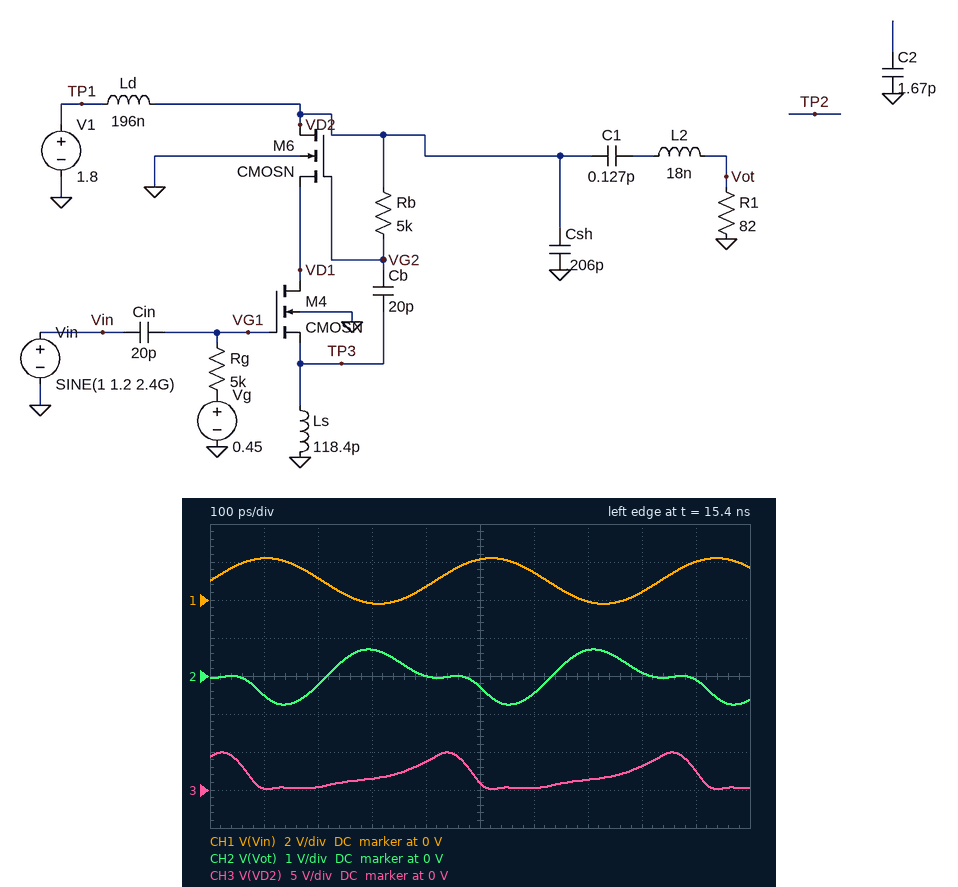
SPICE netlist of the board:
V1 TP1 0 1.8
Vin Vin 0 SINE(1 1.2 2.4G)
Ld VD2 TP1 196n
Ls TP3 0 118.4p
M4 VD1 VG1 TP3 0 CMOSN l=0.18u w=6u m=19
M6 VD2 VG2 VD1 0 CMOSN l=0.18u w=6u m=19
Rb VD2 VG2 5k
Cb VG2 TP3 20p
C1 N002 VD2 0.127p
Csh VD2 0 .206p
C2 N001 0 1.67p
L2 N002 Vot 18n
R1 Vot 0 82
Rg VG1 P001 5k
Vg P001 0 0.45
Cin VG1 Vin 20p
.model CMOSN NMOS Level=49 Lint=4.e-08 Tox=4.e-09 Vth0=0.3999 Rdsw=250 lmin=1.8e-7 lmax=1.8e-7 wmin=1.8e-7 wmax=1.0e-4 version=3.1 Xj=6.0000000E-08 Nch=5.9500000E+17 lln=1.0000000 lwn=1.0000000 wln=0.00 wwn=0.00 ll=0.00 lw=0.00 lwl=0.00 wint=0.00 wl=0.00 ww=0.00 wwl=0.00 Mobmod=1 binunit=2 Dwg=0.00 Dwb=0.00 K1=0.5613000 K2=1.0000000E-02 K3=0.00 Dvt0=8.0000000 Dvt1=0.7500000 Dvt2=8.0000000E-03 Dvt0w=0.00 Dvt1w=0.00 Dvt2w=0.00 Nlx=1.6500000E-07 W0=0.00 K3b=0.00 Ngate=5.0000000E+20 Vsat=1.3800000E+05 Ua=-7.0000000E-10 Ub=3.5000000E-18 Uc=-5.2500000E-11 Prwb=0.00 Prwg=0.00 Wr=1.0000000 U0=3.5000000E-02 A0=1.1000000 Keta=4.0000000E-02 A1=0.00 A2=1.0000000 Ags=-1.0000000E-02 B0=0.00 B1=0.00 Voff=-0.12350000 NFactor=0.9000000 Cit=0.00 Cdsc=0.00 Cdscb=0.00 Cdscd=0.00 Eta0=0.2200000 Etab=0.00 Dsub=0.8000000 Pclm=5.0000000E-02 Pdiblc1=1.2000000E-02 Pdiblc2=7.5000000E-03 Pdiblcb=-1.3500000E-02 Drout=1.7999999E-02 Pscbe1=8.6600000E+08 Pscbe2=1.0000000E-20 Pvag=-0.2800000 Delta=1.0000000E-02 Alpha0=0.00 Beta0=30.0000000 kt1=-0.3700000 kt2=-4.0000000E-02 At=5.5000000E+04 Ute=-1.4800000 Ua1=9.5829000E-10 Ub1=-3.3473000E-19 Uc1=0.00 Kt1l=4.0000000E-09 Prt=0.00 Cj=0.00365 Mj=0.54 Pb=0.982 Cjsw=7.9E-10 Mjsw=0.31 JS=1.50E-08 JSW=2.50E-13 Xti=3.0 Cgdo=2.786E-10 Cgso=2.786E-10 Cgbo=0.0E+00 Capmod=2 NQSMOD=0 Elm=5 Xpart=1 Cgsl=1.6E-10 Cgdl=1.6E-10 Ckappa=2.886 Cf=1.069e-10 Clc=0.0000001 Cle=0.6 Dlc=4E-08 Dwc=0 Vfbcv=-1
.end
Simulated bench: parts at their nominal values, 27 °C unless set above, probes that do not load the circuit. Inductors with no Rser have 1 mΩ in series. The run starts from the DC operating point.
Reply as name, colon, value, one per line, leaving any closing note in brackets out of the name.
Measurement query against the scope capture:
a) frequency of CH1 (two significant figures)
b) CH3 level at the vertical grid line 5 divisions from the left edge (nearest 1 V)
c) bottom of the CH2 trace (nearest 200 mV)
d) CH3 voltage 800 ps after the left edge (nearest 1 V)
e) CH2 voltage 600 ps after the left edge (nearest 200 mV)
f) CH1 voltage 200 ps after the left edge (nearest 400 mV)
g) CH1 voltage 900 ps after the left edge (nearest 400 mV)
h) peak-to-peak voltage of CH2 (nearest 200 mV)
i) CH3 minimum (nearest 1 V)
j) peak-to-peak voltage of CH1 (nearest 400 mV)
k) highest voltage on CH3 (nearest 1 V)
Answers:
frequency of CH1: 2.4 GHz
CH3 level at the vertical grid line 5 divisions from the left edge: 1 V
bottom of the CH2 trace: -800 mV
CH3 voltage 800 ps after the left edge: 3 V
CH2 voltage 600 ps after the left edge: -400 mV
CH1 voltage 200 ps after the left edge: 1.2 V
CH1 voltage 900 ps after the left edge: 2.0 V
peak-to-peak voltage of CH2: 1.4 V
CH3 minimum: 0 V
peak-to-peak voltage of CH1: 2.4 V
highest voltage on CH3: 5 V
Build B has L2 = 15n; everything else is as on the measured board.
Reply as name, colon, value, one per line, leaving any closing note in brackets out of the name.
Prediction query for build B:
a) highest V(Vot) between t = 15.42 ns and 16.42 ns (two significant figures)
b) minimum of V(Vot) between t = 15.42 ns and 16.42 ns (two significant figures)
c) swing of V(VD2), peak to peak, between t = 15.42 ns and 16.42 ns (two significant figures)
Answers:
highest V(Vot) between t = 15.42 ns and 16.42 ns: 720 mV
minimum of V(Vot) between t = 15.42 ns and 16.42 ns: -860 mV
swing of V(VD2), peak to peak, between t = 15.42 ns and 16.42 ns: 5.0 V
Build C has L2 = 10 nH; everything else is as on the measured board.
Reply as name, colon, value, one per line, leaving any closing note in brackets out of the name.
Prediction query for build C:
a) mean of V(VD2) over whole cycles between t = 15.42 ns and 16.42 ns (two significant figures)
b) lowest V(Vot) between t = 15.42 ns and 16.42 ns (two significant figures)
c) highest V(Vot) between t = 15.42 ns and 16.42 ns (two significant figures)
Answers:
mean of V(VD2) over whole cycles between t = 15.42 ns and 16.42 ns: 1.8 V
lowest V(Vot) between t = 15.42 ns and 16.42 ns: -1.3 V
highest V(Vot) between t = 15.42 ns and 16.42 ns: 790 mV
